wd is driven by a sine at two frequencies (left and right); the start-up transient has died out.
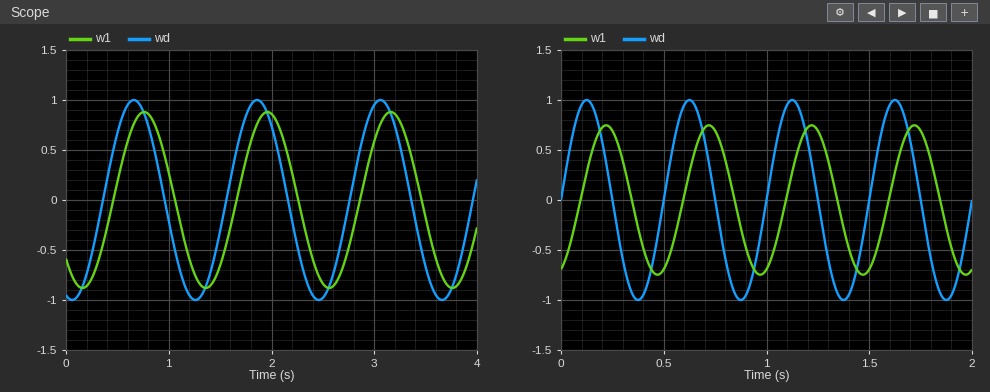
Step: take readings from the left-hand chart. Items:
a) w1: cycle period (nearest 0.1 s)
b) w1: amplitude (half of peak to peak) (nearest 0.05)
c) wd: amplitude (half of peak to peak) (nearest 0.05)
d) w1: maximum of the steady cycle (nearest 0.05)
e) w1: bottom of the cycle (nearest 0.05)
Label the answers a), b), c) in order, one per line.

a) 1.2 s
b) 0.90
c) 1.00
d) 0.90
e) -0.90
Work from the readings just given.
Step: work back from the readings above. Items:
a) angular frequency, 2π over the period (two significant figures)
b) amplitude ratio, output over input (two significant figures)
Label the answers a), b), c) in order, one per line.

a) 5.2 rad/s
b) 0.90
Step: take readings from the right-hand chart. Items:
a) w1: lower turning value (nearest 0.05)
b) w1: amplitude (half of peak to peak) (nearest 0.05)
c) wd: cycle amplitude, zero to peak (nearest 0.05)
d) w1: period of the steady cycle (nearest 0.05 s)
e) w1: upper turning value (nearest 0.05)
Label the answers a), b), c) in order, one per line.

a) -0.75
b) 0.75
c) 1.00
d) 0.50 s
e) 0.75
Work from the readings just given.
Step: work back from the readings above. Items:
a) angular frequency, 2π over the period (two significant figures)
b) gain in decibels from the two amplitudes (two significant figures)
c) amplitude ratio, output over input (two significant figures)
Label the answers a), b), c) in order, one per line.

a) 13 rad/s
b) -2.5 dB
c) 0.75
